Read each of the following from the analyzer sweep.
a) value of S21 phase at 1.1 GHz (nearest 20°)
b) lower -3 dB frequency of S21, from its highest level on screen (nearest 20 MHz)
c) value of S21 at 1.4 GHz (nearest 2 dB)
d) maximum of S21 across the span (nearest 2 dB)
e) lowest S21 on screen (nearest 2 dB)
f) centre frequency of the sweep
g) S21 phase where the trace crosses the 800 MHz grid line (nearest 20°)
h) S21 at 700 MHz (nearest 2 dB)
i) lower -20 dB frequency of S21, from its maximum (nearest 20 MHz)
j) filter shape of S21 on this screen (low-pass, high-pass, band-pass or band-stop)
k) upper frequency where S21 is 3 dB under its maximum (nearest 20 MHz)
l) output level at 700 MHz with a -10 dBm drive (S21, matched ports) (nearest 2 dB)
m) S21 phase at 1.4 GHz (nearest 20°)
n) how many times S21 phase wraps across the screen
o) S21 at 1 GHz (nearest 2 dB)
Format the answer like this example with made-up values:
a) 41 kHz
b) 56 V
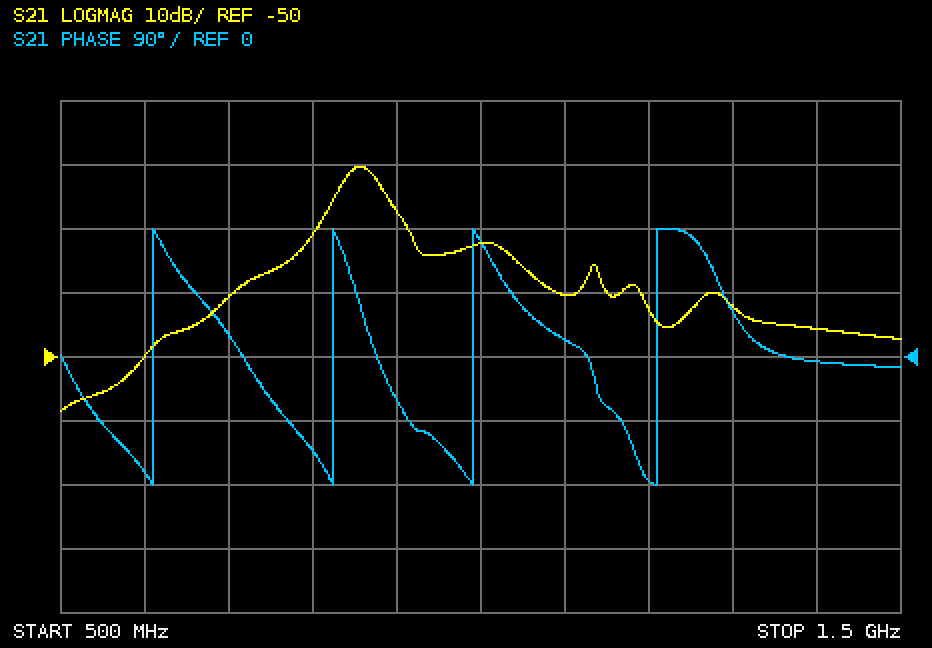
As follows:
a) 20°
b) 840 MHz
c) -46 dB
d) -20 dB
e) -58 dB
f) 1 GHz
g) -140°
h) -40 dB
i) 700 MHz
j) band-pass
k) 880 MHz
l) -50 dBm
m) 0°
n) 4
o) -32 dB
